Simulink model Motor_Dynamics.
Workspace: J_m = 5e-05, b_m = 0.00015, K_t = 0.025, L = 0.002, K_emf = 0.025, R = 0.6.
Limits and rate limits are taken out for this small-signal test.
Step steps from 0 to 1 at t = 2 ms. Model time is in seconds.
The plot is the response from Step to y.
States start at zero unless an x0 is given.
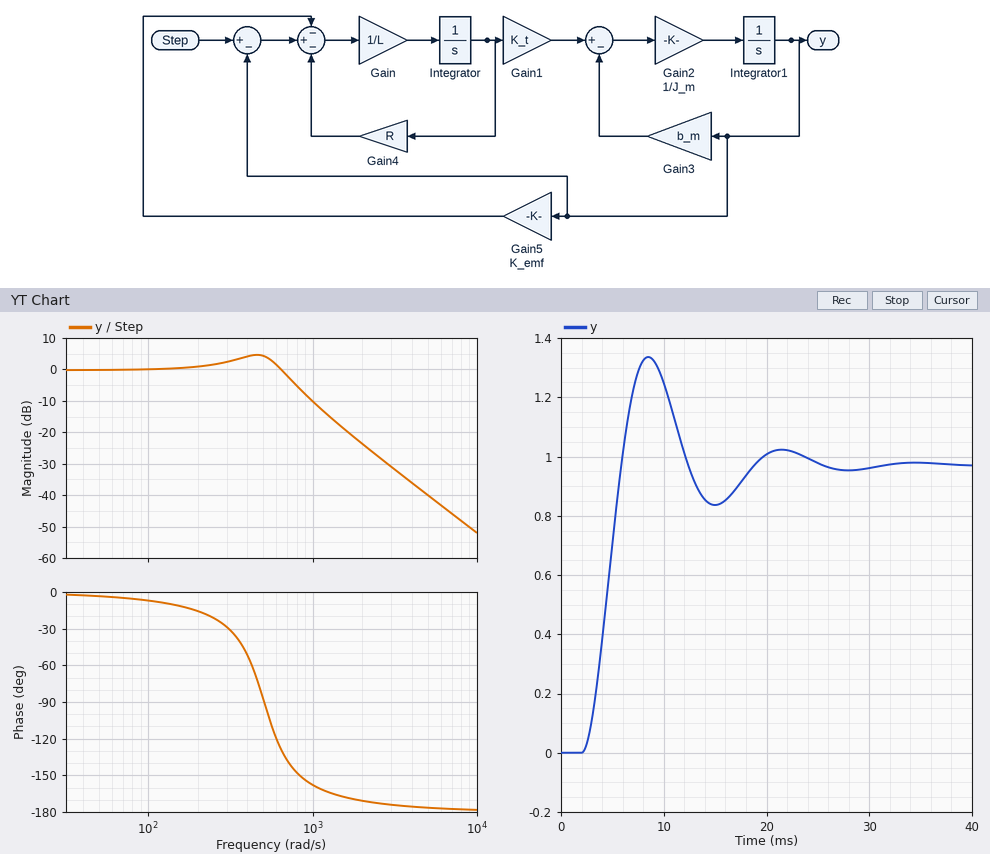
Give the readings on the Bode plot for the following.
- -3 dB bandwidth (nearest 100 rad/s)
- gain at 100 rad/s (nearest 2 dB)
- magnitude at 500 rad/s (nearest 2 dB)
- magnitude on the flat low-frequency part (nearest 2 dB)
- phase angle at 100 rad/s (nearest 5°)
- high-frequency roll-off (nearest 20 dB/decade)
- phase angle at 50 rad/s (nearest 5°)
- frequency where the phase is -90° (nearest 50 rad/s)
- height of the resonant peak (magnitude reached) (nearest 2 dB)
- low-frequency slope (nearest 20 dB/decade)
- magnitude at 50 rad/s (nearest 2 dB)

700 rad/s
0 dB
4 dB
0 dB
-5°
-40 dB/decade
-5°
500 rad/s
4 dB
0 dB/decade
0 dB
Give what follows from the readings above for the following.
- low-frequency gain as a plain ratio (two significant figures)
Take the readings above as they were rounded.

1.0
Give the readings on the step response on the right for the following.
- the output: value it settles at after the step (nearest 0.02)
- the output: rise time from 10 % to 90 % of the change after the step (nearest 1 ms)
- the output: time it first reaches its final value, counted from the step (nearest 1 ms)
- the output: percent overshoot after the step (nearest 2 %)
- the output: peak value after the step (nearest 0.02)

0.98
3 ms
4 ms
38 %
1.34
